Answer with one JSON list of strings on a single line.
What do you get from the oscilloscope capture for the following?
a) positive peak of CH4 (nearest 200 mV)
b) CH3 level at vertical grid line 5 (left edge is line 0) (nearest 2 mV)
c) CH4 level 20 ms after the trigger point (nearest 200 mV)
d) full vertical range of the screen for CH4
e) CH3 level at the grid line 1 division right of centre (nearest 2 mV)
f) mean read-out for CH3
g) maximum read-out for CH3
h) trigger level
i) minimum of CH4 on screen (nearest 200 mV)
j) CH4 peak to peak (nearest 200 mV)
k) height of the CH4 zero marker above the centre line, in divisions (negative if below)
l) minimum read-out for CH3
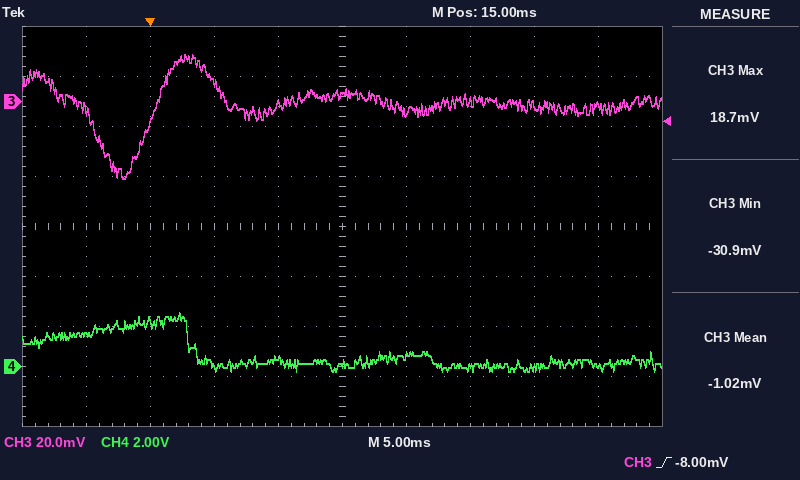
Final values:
["2.2 V", "2 mV", "400 mV", "16 V", "-4 mV", "-1.02 mV", "18.7 mV", "-8.00 mV", "-200 mV", "2.4 V", "-2.8 div", "-30.9 mV"]
